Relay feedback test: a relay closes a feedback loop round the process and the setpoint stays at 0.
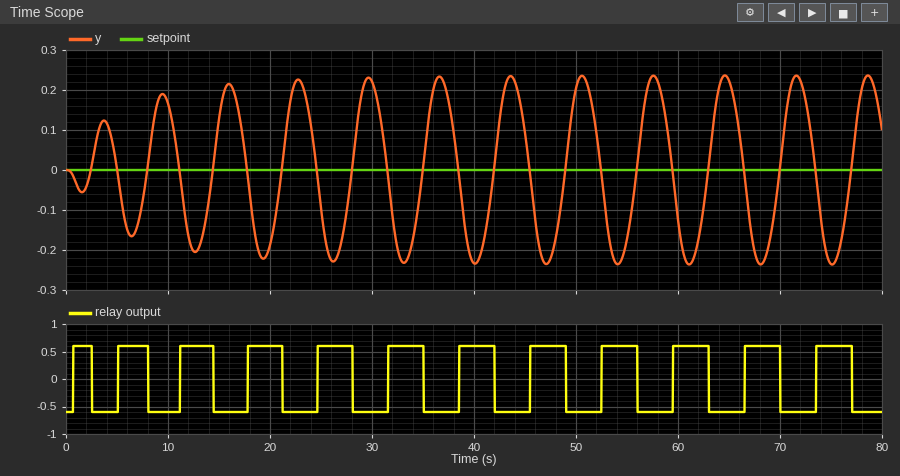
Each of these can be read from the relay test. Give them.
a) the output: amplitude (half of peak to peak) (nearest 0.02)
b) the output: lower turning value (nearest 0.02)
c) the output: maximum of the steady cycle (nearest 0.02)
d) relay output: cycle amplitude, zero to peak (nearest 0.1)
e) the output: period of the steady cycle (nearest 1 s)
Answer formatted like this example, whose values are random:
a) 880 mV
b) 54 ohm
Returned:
a) 0.24
b) -0.24
c) 0.24
d) 0.6
e) 7 s
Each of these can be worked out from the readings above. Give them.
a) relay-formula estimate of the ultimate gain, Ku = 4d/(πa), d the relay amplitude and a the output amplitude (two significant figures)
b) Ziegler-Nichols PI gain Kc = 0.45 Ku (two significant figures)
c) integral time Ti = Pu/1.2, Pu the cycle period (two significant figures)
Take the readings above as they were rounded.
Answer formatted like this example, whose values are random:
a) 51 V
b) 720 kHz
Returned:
a) 3.2
b) 1.4
c) 5.8 s
